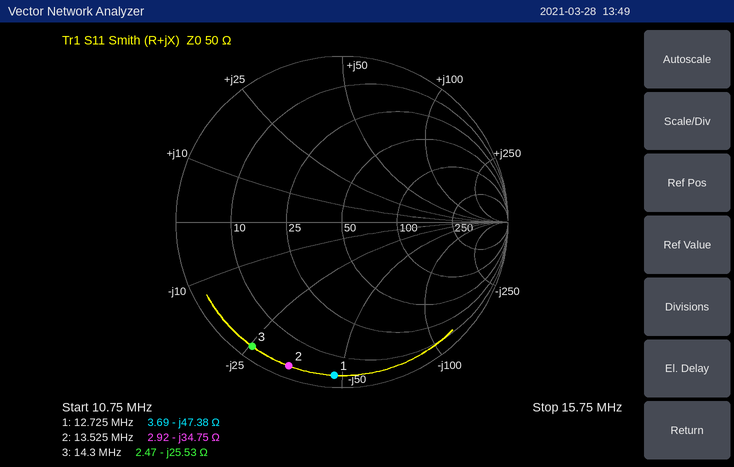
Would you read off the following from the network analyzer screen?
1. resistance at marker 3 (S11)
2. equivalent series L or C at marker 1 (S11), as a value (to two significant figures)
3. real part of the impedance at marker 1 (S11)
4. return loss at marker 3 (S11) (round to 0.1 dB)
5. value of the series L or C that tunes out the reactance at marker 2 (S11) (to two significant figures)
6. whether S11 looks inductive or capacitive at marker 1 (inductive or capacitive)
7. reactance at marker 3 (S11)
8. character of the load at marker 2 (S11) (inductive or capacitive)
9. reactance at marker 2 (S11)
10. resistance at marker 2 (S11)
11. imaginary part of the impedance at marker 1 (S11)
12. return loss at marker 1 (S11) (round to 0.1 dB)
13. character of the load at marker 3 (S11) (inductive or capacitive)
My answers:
2.47 Ω
260 pF
3.69 Ω
0.7 dB
410 nH
capacitive
-25.53 Ω
capacitive
-34.75 Ω
2.92 Ω
-47.38 Ω
0.7 dB
capacitive
